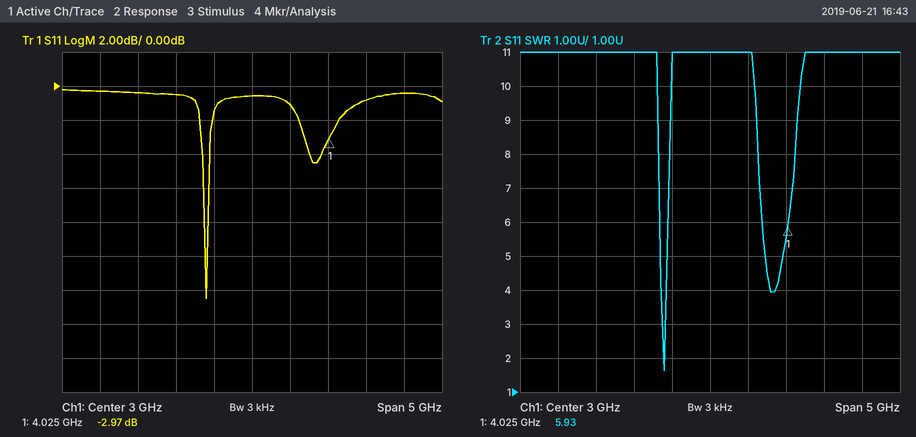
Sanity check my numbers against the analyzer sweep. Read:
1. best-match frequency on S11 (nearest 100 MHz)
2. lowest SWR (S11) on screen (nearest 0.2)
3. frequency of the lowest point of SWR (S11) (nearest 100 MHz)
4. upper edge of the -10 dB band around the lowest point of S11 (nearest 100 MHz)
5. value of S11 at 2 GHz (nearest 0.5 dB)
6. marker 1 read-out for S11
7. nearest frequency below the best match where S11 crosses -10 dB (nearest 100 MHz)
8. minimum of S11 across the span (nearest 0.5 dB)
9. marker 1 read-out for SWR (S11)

2.4 GHz
1.6
2.4 GHz
2.4 GHz
-0.5 dB
-2.97 dB
2.4 GHz
-12.5 dB
5.93
